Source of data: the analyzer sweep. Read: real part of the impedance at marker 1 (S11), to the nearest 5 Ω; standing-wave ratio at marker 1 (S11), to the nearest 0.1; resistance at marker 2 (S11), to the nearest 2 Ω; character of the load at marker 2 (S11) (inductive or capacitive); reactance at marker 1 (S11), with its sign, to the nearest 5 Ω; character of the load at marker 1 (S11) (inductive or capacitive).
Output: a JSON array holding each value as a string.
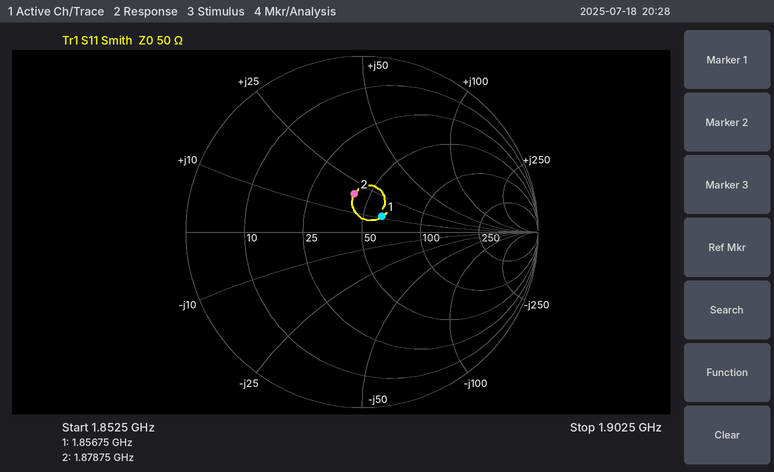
["60 Ω", "1.3", "42 Ω", "inductive", "+10 Ω", "inductive"]
